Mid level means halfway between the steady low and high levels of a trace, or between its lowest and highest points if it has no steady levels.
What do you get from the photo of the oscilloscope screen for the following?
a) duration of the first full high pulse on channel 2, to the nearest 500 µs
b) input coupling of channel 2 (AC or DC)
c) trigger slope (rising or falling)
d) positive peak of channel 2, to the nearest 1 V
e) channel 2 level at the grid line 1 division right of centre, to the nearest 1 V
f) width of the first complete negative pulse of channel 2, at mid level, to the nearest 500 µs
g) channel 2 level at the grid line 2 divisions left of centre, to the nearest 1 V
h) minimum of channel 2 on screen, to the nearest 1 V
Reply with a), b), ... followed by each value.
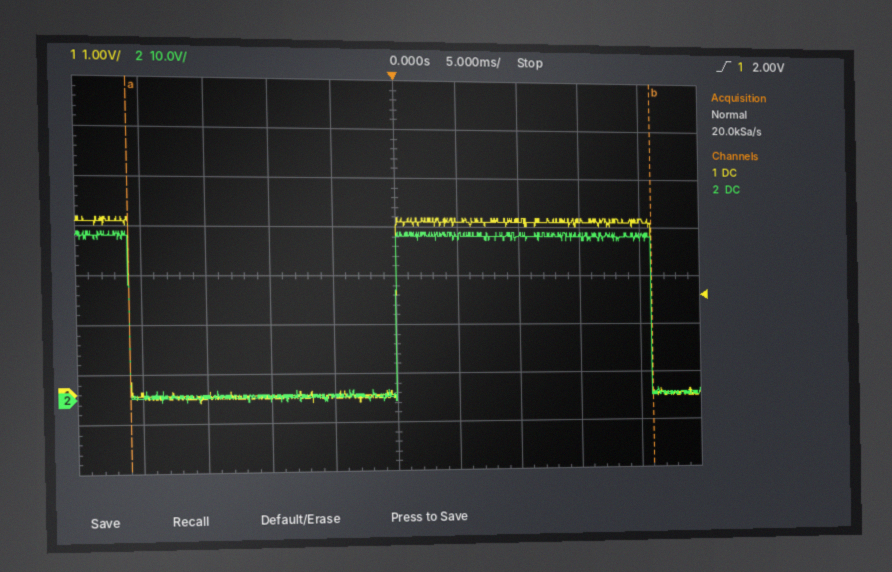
a) 21.0 ms
b) DC
c) rising
d) 34 V
e) 33 V
f) 21.0 ms
g) 0 V
h) -1 V
